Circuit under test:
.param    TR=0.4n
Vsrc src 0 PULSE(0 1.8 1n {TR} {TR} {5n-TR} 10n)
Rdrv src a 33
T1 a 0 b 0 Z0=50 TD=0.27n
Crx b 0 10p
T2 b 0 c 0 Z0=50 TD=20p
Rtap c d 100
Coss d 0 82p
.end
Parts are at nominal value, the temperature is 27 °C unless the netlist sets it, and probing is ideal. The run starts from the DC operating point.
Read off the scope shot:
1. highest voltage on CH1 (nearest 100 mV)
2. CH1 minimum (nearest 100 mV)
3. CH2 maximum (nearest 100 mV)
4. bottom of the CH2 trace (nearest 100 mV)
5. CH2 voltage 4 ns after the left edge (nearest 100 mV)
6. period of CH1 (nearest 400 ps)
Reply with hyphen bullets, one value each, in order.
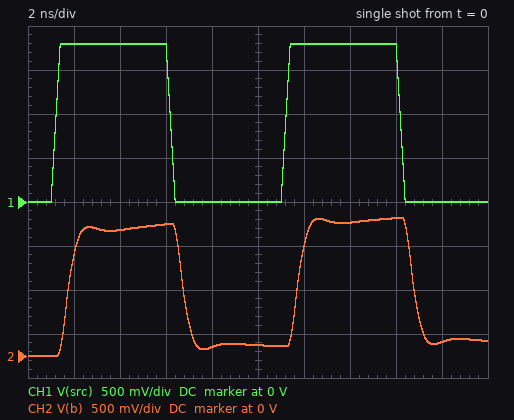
- 1.8 V
- 0 V
- 1.6 V
- 0 V
- 1.4 V
- 10.0 ns
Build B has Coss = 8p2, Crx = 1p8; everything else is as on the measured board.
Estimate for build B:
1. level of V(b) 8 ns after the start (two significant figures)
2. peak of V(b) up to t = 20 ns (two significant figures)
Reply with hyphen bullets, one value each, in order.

- 89 mV
- 1.8 V
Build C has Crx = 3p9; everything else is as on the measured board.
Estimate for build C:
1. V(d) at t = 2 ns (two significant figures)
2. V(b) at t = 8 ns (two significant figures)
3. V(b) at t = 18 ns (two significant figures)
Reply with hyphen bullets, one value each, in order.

- 67 mV
- 150 mV
- 210 mV
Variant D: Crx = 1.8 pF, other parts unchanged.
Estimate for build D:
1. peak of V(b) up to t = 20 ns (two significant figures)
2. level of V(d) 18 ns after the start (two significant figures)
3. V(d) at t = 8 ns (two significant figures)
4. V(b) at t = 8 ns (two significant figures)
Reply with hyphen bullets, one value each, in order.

- 1.6 V
- 810 mV
- 580 mV
- 150 mV
